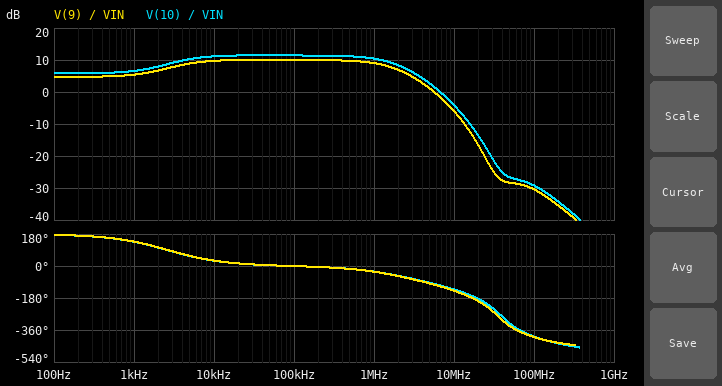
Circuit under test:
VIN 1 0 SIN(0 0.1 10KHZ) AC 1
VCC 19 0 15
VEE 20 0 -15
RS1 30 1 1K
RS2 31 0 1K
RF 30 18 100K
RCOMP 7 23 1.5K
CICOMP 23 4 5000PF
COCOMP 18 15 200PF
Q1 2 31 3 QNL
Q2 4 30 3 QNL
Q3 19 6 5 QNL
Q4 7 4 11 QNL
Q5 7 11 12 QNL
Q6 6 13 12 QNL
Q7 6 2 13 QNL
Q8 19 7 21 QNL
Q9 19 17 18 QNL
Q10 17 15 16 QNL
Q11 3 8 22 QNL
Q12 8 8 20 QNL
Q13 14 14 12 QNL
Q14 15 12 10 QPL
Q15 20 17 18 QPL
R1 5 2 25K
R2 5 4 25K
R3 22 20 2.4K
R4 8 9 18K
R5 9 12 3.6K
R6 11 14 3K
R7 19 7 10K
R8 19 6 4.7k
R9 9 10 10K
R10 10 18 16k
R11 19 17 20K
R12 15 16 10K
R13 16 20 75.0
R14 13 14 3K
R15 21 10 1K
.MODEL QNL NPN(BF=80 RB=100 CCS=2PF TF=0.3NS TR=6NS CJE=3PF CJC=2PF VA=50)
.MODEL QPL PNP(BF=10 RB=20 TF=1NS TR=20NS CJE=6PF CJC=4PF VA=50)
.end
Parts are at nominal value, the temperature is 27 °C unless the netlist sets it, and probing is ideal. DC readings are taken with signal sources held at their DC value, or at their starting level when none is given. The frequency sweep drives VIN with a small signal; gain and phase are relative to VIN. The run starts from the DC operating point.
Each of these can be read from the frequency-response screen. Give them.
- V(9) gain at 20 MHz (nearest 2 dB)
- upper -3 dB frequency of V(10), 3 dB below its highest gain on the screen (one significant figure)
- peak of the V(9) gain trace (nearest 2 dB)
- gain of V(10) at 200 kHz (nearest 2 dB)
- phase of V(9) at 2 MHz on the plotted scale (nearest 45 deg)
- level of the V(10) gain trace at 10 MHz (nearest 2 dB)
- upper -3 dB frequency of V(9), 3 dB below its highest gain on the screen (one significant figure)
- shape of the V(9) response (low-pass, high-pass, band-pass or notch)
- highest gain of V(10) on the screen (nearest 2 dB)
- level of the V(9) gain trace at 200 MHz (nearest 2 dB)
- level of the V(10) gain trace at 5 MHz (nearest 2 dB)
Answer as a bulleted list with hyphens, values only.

- -16 dB
- 2 MHz
- 10 dB
- 12 dB
- -45 deg
- -4 dB
- 2 MHz
- low-pass
- 12 dB
- -36 dB
- 2 dB
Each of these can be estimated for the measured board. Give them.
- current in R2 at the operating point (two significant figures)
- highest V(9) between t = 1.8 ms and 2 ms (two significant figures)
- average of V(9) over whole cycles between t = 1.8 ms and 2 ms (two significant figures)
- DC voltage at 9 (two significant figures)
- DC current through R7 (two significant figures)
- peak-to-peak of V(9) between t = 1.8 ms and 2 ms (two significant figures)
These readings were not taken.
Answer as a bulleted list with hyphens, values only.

- 20 µA
- 7.1 V
- 6.9 V
- 6.9 V
- 260 µA
- 350 mV
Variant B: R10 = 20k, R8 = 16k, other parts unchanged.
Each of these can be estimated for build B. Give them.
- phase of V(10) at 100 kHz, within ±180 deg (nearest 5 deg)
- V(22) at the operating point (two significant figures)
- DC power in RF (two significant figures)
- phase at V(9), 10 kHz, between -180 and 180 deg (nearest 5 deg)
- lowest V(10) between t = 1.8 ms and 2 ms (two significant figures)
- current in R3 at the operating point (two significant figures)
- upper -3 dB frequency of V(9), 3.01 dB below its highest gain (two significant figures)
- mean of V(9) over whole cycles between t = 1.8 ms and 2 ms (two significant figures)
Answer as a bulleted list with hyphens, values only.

- 150 deg
- -15 V
- 170 nW
- 145 deg
- 8.6 V
- 39 µA
- 4.7 kHz
- 5.3 V
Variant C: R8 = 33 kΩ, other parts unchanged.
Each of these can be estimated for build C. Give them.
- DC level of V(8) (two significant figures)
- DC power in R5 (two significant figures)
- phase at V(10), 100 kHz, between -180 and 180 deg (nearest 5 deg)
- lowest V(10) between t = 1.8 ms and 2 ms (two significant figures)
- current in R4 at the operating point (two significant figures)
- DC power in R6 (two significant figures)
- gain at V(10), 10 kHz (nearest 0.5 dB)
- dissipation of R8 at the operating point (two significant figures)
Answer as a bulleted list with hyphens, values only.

- -14 V
- 1.8 mW
- 170 deg
- 7.6 V
- 1.0 mA
- 1.6 µW
- 9.0 dB
- 870 µW
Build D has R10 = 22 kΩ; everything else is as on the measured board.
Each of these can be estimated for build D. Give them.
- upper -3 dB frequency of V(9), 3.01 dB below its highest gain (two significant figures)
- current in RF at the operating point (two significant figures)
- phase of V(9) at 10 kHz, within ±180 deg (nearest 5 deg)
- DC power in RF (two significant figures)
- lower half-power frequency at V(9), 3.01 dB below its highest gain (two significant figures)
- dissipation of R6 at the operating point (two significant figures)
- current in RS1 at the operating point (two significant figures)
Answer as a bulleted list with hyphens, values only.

- 1.9 MHz
- 1.8 µA
- 35 deg
- 310 nW
- 3.9 kHz
- 760 nW
- 1.6 µA
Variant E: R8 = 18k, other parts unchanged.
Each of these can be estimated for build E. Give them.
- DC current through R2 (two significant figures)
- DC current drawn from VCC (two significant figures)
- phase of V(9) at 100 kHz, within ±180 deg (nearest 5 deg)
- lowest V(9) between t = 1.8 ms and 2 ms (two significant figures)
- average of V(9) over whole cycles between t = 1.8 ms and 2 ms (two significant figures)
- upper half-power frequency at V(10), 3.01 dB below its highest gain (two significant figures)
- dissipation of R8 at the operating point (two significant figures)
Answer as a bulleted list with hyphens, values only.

- 19 µA
- 2.5 mA
- 160 deg
- 5.0 V
- 5.1 V
- 3.8 kHz
- 1.2 mW
